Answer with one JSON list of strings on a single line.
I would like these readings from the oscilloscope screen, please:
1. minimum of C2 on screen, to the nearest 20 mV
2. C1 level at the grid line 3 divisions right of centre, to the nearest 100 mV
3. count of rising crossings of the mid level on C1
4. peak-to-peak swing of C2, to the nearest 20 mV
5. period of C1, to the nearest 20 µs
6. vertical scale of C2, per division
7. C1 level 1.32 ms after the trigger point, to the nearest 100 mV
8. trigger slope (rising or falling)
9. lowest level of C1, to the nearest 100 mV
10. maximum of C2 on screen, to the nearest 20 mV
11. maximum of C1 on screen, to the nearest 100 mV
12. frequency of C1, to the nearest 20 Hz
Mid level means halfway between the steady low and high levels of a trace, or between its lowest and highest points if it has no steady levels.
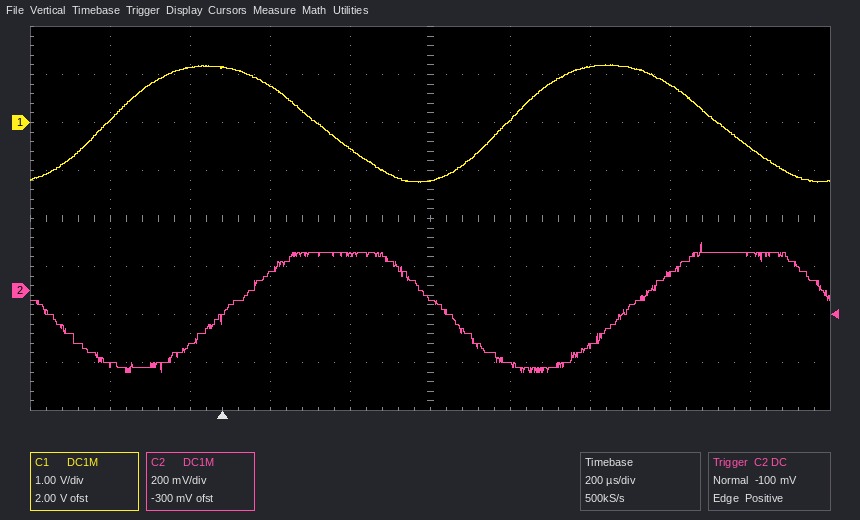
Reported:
["-340 mV", "800 mV", "2", "540 mV", "1.00 ms", "200 mV", "-500 mV", "rising", "-1.2 V", "200 mV", "1.2 V", "1.00 kHz"]
